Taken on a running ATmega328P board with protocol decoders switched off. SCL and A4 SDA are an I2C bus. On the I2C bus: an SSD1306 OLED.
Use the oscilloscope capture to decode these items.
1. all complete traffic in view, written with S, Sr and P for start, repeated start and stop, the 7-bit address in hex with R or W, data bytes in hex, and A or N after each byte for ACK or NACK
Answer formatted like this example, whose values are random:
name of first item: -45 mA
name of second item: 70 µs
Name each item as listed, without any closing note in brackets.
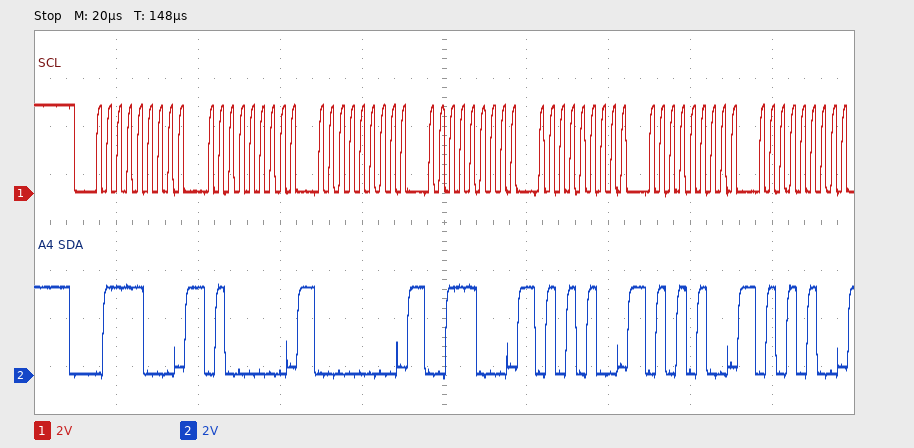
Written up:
all complete traffic in view, written with S, Sr and P for start, repeated start and stop, the 7-bit address in hex with R or W, data bytes in hex, and A or N after each byte for ACK or NACK: S 3CW A 40 A 00 A 38 A 54 A 54 A 54 A
